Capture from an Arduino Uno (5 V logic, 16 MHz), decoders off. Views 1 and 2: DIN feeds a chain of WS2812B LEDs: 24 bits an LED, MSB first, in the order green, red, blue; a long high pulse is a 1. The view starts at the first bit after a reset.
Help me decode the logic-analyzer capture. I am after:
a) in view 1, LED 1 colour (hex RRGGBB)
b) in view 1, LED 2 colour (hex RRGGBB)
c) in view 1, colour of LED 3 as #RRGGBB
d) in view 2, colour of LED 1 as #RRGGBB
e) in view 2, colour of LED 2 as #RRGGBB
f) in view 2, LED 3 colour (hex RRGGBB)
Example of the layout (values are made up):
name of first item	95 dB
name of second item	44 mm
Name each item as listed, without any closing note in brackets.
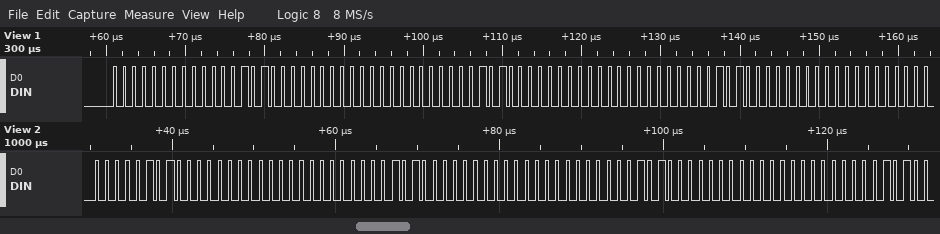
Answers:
in view 1, LED 1 colour	#050000
in view 1, LED 2 colour	#050000
in view 1, colour of LED 3 as #RRGGBB	#050000
in view 2, colour of LED 1 as #RRGGBB	#000500
in view 2, colour of LED 2 as #RRGGBB	#000500
in view 2, LED 3 colour	#000500
